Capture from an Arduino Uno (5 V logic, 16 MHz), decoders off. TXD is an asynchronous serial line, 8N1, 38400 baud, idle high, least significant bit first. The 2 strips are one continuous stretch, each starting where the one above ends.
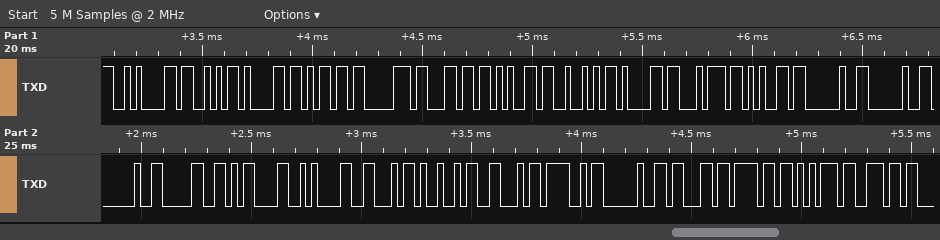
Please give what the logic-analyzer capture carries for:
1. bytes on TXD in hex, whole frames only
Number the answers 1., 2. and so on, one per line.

1. 0x0A 0x53 0x61 0x6D 0x70 0x6C 0x65 0x52 0x61 0x74 0x65 0x20 0x20 0x20 0x30 0x0D 0x0A 0x46 0x49 0x46 0x4F 0x20 0x63 0x6F 0x75 0x6E
